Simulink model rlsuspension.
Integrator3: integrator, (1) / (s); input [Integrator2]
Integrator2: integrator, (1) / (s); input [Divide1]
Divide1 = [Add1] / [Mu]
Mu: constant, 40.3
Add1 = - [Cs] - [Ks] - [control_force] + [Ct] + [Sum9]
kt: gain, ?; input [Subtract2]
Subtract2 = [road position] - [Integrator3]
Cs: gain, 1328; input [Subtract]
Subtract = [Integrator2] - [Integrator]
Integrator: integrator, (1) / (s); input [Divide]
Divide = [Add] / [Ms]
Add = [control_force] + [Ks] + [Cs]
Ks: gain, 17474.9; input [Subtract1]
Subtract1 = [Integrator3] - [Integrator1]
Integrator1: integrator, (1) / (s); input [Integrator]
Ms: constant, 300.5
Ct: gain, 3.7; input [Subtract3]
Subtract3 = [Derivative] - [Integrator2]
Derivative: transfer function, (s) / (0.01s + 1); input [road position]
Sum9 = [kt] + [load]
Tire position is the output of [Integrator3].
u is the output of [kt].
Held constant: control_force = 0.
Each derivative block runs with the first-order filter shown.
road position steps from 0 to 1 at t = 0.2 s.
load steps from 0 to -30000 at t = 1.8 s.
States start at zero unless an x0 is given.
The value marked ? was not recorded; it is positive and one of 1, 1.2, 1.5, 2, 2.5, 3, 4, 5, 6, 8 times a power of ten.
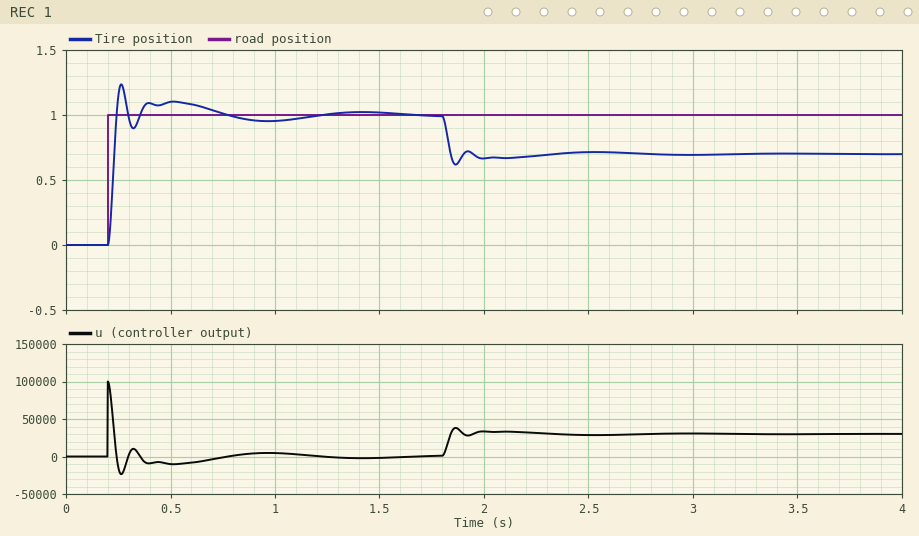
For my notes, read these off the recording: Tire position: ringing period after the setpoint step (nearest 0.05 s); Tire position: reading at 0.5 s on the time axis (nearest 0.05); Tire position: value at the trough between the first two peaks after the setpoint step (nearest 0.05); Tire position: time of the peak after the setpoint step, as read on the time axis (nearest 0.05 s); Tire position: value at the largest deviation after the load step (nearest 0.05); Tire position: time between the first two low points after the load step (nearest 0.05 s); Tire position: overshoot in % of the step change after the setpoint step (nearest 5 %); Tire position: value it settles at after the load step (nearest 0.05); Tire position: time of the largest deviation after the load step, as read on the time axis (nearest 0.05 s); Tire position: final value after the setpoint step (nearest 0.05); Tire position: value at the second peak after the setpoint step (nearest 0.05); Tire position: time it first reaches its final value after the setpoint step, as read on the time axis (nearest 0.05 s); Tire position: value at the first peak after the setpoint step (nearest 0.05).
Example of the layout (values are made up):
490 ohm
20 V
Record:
0.25 s
1.10
0.90
0.25 s
0.60
0.15 s
25 %
0.70
1.85 s
1.00
1.10
0.25 s
1.25
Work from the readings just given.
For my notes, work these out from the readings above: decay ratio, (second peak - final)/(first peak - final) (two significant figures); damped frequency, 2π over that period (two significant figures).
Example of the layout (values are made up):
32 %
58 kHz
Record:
0.40
25 rad/s
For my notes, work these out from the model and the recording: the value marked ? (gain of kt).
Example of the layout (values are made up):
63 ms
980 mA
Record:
100000
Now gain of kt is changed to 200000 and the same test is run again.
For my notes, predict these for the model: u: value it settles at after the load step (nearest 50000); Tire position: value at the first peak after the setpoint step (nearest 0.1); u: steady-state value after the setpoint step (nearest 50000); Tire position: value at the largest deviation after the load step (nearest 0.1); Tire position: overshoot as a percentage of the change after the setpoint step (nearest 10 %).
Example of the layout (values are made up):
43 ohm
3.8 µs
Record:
50000
1.4
0
0.8
40 %
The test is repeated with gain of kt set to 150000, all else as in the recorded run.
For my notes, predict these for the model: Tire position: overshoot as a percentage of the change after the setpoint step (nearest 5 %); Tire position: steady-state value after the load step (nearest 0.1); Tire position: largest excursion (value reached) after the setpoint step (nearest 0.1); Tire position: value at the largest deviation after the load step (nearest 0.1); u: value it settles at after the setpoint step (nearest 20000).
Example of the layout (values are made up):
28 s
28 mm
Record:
35 %
0.8
1.3
0.7
0
